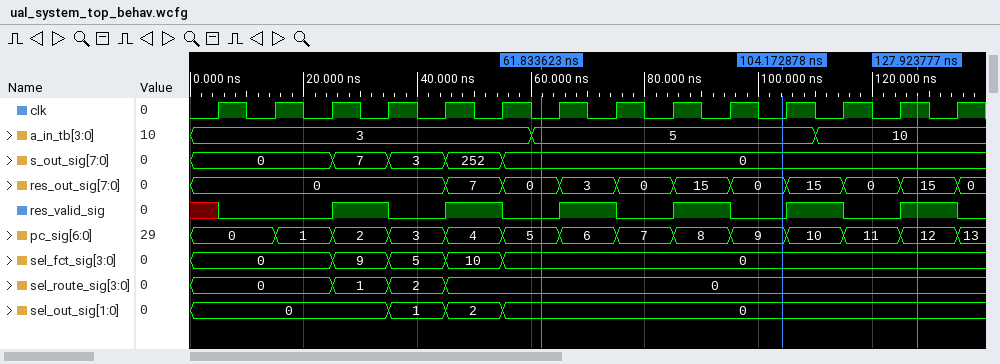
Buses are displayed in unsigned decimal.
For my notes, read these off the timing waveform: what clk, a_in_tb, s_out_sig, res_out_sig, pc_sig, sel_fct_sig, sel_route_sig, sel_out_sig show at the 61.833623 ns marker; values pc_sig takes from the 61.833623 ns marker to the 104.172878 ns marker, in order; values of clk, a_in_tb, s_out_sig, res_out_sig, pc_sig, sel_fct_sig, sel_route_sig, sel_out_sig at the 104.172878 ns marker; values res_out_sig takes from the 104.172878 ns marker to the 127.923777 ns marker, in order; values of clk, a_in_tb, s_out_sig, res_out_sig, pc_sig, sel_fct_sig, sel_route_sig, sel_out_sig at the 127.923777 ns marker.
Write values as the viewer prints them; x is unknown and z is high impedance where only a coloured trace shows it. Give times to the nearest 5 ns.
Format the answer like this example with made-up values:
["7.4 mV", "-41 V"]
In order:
["clk=0, a_in_tb=5, s_out_sig=0, res_out_sig=0, pc_sig=5, sel_fct_sig=0, sel_route_sig=0, sel_out_sig=0", "5, 6, 7, 8, 9", "clk=0, a_in_tb=5, s_out_sig=0, res_out_sig=0, pc_sig=9, sel_fct_sig=0, sel_route_sig=0, sel_out_sig=0", "0, 15, 0, 15", "clk=1, a_in_tb=10, s_out_sig=0, res_out_sig=15, pc_sig=12, sel_fct_sig=0, sel_route_sig=0, sel_out_sig=0"]
